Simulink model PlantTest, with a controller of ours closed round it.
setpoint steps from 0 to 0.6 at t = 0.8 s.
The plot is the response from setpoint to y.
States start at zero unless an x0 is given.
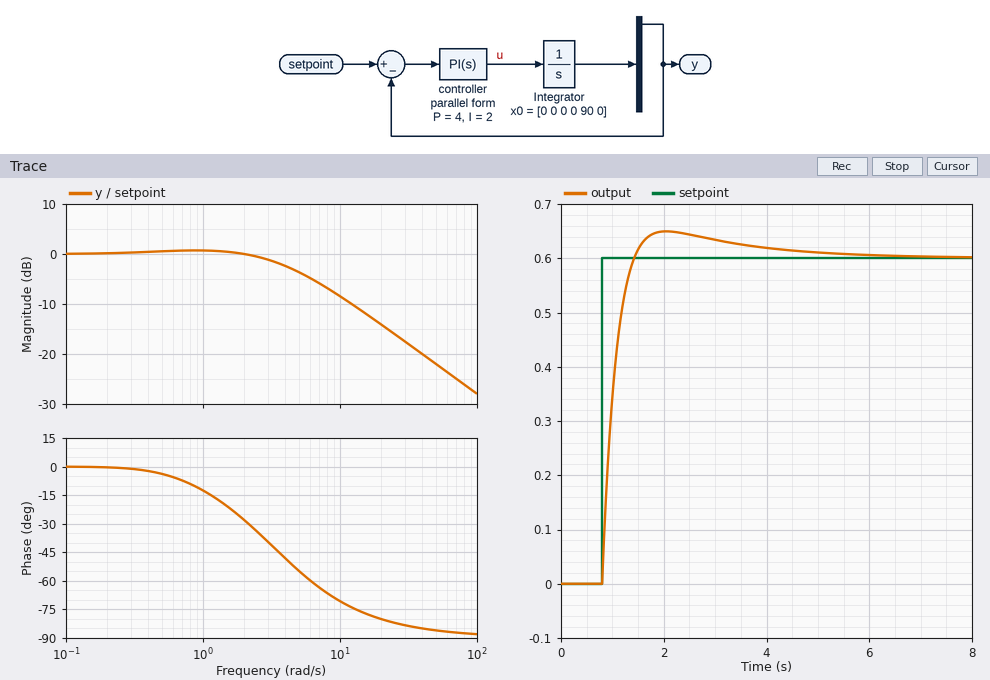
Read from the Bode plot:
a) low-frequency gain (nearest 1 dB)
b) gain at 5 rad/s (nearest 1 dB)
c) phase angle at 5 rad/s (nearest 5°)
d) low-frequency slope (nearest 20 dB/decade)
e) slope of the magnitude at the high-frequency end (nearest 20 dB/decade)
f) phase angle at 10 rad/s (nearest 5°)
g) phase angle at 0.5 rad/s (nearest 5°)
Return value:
0 dB
-4 dB
-55°
0 dB/decade
-20 dB/decade
-70°
-5°
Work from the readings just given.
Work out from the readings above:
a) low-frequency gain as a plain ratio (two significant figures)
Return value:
1.0
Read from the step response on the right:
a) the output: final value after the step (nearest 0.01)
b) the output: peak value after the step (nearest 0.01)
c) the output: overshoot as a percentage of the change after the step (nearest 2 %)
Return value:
0.60
0.65
8 %
